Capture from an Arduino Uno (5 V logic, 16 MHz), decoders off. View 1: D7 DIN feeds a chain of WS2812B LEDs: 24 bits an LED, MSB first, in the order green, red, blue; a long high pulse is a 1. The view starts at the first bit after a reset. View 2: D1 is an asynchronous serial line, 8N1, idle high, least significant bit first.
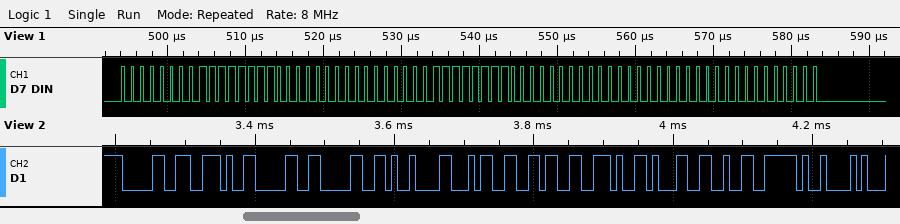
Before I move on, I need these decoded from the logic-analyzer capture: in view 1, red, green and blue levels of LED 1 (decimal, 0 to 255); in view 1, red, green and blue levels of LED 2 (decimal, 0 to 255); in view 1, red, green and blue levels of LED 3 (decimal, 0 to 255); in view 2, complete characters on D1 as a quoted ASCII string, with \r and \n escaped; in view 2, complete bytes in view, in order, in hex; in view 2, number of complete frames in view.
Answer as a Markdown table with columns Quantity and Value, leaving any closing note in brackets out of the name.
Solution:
| Quantity | Value |
|---|---|
| in view 1, red, green and blue levels of LED 1 | 255, 0, 0 |
| in view 1, red, green and blue levels of LED 2 | 255, 0, 0 |
| in view 1, red, green and blue levels of LED 3 | 0, 0, 0 |
| in view 2, complete characters on D1 as a quoted ASCII string, with \r and \n escaped | "0.00\t46.12\t" |
| in view 2, complete bytes in view, in order, in hex | 30 2E 30 30 09 34 36 2E 31 32 09 |
| in view 2, number of complete frames in view | 11 |
